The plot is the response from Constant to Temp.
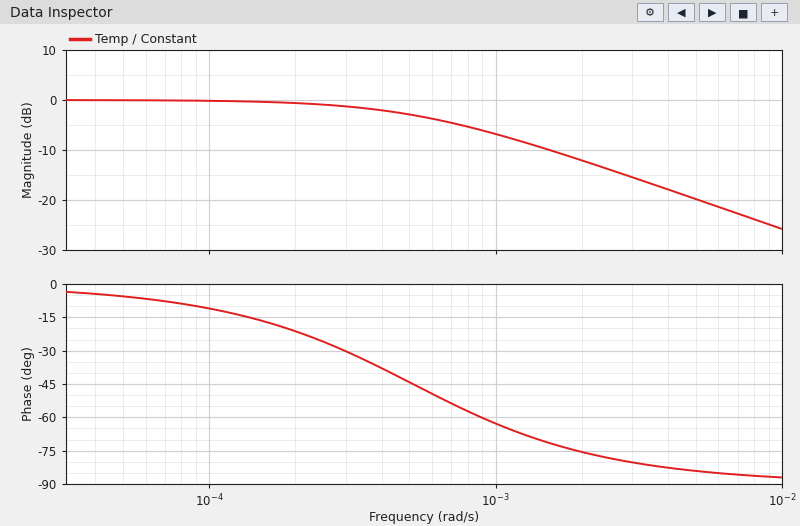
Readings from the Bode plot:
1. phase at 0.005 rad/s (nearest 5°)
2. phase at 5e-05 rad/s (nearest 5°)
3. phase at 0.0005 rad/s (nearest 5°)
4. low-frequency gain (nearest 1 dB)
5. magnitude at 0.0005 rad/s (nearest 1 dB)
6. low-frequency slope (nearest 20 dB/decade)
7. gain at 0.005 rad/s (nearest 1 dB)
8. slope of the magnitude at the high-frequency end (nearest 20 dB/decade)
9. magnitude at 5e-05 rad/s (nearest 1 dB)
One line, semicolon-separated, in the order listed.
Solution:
-85°; -5°; -45°; 0 dB; -3 dB; 0 dB/decade; -20 dB; -20 dB/decade; 0 dB
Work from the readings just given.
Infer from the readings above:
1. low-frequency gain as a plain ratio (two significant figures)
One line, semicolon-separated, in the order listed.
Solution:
1.0
